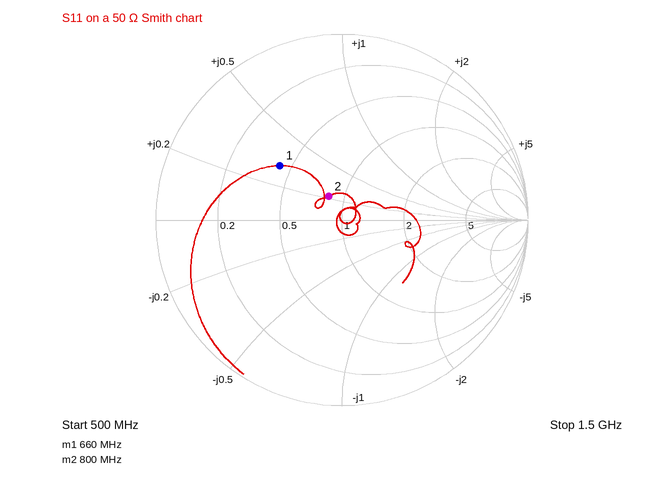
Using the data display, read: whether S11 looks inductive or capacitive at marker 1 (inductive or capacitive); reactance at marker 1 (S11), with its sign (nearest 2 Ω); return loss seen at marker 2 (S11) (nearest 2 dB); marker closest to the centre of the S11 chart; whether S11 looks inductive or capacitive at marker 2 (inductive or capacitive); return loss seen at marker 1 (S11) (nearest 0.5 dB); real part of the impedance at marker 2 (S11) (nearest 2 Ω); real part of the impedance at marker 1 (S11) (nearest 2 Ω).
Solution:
inductive
+16 Ω
16 dB
marker 2
inductive
7.0 dB
42 Ω
22 Ω
